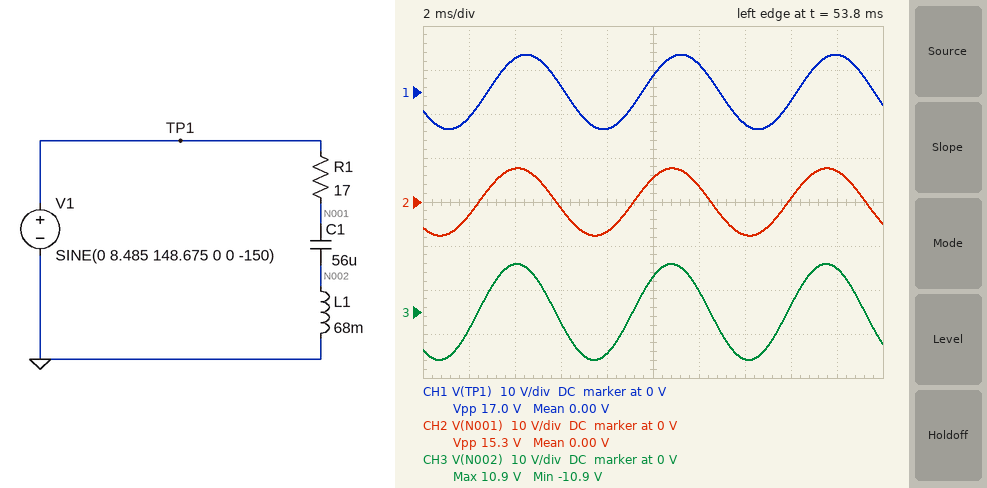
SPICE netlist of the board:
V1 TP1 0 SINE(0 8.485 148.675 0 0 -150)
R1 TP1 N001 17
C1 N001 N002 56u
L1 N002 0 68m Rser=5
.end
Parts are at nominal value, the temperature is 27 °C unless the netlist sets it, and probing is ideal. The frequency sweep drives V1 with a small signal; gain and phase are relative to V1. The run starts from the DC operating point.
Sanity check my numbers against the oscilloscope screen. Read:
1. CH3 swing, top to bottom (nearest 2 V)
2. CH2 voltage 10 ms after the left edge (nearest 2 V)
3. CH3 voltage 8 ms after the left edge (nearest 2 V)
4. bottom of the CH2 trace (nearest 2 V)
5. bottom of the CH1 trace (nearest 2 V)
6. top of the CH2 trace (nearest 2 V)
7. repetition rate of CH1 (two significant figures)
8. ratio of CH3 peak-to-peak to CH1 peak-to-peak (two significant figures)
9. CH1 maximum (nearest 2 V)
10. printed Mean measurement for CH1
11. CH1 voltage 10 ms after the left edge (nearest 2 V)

22 V
6 V
-10 V
-8 V
-8 V
8 V
150 Hz
1.3
8 V
0.00 V
4 V
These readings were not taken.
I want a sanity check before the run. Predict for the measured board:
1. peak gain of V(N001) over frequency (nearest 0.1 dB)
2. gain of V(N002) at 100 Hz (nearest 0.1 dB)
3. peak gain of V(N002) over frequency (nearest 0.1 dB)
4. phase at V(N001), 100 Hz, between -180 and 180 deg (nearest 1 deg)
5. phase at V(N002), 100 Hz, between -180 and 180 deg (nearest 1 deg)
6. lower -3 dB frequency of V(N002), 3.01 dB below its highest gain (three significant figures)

0 dB
4.3 dB
4.5 dB
38 deg
50 deg
68.8 Hz
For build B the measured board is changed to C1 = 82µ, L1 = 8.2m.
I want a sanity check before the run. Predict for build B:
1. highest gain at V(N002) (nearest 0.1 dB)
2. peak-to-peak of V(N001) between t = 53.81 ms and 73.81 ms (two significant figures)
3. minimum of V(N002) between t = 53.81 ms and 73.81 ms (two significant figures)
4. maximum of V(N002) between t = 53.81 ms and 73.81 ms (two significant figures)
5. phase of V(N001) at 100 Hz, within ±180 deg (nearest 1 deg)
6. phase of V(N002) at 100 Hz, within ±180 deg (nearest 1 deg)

0 dB
5.5 V
-3.4 V
3.4 V
-38 deg
79 deg
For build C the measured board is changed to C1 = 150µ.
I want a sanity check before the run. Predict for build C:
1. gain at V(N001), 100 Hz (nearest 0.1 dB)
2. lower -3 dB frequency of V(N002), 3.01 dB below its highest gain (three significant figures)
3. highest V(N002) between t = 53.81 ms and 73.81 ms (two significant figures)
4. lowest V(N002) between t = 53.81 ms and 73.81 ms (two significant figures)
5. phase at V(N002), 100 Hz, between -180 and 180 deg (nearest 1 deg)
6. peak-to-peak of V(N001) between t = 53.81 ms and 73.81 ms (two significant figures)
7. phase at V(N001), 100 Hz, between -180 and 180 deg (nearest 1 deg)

-1.6 dB
42.2 Hz
8.9 V
-8.9 V
28 deg
16 V
26 deg
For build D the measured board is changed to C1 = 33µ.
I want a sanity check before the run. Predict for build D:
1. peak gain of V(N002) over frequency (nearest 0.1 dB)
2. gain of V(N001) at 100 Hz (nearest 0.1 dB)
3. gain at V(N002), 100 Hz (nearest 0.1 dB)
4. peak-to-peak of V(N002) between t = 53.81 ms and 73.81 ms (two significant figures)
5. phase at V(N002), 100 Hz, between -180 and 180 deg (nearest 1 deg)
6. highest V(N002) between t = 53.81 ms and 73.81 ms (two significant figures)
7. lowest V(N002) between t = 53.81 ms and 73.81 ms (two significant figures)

6.6 dB
-9.7 dB
5.6 dB
28 V
97 deg
14 V
-14 V
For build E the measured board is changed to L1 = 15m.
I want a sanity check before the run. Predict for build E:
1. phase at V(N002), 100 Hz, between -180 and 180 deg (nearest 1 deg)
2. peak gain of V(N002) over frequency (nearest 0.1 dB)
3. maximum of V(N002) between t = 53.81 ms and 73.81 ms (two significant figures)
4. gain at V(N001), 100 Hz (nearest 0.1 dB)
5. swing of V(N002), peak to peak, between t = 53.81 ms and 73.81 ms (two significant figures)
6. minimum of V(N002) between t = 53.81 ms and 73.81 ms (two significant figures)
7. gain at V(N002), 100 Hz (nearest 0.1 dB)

103 deg
0.1 dB
5.6 V
-3.4 dB
11 V
-5.6 V
-8.7 dB
